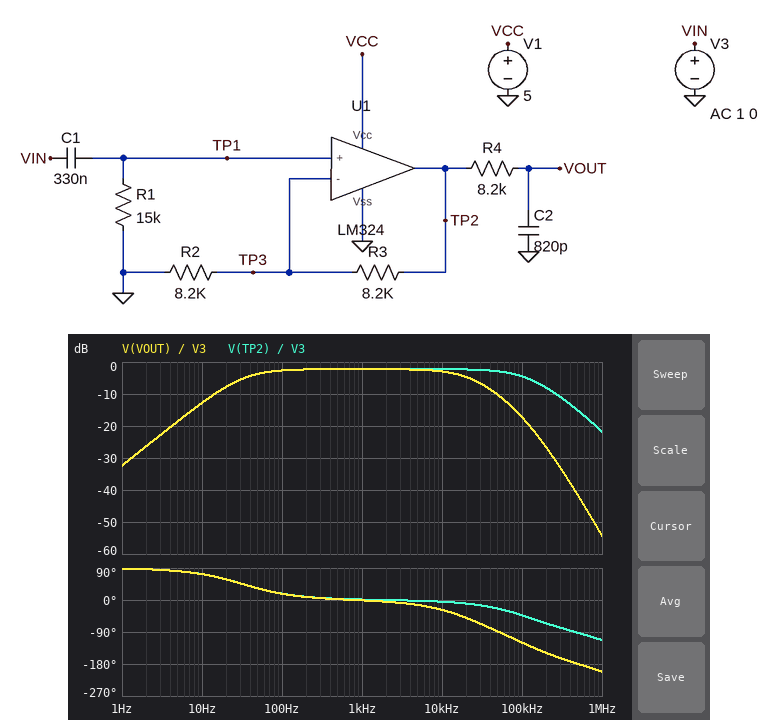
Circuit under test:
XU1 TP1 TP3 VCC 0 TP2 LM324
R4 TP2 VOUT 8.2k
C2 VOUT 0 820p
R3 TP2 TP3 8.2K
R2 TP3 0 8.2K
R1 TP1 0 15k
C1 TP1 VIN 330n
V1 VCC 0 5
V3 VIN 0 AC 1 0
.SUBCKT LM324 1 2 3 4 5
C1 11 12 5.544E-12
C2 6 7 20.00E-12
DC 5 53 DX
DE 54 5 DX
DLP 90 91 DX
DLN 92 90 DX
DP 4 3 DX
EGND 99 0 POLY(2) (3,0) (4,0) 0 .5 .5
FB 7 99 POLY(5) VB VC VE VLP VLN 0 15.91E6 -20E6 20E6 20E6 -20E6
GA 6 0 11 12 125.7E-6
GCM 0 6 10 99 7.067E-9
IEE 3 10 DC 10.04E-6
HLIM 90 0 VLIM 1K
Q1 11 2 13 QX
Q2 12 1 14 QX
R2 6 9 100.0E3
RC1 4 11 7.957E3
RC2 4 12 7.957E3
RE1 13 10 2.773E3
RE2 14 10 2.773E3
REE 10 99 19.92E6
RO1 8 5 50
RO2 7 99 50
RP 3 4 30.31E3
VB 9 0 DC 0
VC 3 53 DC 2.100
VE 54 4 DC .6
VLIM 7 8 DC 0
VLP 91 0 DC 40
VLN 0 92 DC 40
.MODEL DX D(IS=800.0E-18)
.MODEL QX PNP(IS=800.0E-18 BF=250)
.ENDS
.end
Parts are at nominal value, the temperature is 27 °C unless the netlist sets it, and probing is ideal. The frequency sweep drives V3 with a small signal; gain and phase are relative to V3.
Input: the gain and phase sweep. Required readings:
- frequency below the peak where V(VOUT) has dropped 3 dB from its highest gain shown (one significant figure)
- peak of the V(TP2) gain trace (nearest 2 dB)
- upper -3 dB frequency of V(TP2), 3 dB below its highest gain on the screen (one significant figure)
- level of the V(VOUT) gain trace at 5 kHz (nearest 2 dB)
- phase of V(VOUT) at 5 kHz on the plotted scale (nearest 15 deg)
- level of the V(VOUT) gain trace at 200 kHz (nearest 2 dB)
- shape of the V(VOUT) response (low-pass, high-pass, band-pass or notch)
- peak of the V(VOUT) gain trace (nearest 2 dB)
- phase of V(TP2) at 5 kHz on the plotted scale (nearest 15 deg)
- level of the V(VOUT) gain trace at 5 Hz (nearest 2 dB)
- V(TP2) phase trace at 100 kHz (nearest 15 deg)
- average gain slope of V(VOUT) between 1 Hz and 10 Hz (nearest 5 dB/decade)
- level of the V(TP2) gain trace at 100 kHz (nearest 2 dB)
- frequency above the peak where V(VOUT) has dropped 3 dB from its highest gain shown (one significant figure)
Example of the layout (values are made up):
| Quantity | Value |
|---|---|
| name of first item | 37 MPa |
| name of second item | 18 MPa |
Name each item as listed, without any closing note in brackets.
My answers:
| Quantity | Value |
|---|---|
| frequency below the peak where V(VOUT) has dropped 3 dB from its highest gain shown | 30 Hz |
| peak of the V(TP2) gain trace | -2 dB |
| upper -3 dB frequency of V(TP2), 3 dB below its highest gain on the screen | 100 kHz |
| level of the V(VOUT) gain trace at 5 kHz | -2 dB |
| phase of V(VOUT) at 5 kHz on the plotted scale | -15 deg |
| level of the V(VOUT) gain trace at 200 kHz | -26 dB |
| shape of the V(VOUT) response | band-pass |
| peak of the V(VOUT) gain trace | -2 dB |
| phase of V(TP2) at 5 kHz on the plotted scale | 0 deg |
| level of the V(VOUT) gain trace at 5 Hz | -18 dB |
| V(TP2) phase trace at 100 kHz | -45 deg |
| average gain slope of V(VOUT) between 1 Hz and 10 Hz | 20 dB/decade |
| level of the V(TP2) gain trace at 100 kHz | -4 dB |
| frequency above the peak where V(VOUT) has dropped 3 dB from its highest gain shown | 20 kHz |
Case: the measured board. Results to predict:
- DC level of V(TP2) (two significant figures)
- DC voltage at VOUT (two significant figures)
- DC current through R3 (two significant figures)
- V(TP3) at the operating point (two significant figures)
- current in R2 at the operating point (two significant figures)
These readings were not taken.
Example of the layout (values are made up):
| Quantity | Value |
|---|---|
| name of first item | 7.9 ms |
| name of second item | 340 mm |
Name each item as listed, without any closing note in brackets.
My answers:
| Quantity | Value |
|---|---|
| DC level of V(TP2) | 41 mV |
| DC voltage at VOUT | 41 mV |
| DC current through R3 | 2.5 µA |
| V(TP3) at the operating point | 20 mV |
| current in R2 at the operating point | 2.5 µA |
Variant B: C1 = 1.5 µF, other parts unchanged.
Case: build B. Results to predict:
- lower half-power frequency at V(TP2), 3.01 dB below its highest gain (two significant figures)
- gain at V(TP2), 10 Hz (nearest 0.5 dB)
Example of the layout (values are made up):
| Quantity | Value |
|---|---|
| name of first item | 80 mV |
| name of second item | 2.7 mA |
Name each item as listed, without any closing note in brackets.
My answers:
| Quantity | Value |
|---|---|
| lower half-power frequency at V(TP2), 3.01 dB below its highest gain | 7.1 Hz |
| gain at V(TP2), 10 Hz | -4.0 dB |
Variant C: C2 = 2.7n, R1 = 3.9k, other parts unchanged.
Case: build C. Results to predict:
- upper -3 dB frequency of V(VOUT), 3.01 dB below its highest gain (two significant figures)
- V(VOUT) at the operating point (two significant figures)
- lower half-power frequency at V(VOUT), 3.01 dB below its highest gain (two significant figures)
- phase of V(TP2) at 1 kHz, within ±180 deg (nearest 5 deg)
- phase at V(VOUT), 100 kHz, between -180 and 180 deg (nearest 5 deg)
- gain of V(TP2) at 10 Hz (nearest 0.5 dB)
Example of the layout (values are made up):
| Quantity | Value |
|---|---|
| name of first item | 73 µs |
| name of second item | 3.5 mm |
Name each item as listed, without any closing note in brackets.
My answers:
| Quantity | Value |
|---|---|
| upper -3 dB frequency of V(VOUT), 3.01 dB below its highest gain | 7.4 kHz |
| V(VOUT) at the operating point | 40 mV |
| lower half-power frequency at V(VOUT), 3.01 dB below its highest gain | 120 Hz |
| phase of V(TP2) at 1 kHz, within ±180 deg | 5 deg |
| phase at V(VOUT), 100 kHz, between -180 and 180 deg | -130 deg |
| gain of V(TP2) at 10 Hz | -24.0 dB |
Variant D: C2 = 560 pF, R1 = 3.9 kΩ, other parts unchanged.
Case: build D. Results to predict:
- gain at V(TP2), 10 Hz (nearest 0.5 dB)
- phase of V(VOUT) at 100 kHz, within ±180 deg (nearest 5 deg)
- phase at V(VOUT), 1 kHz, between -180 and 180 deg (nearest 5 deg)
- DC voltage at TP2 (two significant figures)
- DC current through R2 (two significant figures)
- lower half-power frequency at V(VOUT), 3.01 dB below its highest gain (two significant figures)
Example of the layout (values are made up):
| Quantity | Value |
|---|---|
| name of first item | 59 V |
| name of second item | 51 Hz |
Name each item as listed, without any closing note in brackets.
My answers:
| Quantity | Value |
|---|---|
| gain at V(TP2), 10 Hz | -24.0 dB |
| phase of V(VOUT) at 100 kHz, within ±180 deg | -115 deg |
| phase at V(VOUT), 1 kHz, between -180 and 180 deg | 5 deg |
| DC voltage at TP2 | 40 mV |
| DC current through R2 | 2.5 µA |
| lower half-power frequency at V(VOUT), 3.01 dB below its highest gain | 120 Hz |
